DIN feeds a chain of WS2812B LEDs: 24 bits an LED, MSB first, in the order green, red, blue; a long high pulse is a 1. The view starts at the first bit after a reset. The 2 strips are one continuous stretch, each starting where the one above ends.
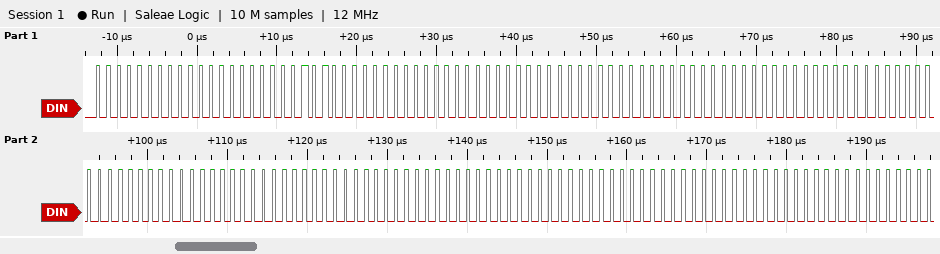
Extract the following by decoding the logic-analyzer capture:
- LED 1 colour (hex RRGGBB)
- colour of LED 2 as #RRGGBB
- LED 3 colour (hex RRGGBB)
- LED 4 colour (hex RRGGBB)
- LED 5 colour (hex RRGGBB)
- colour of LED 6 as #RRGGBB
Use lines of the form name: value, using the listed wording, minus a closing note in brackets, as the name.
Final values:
LED 1 colour: #00000A
colour of LED 2 as #RRGGBB: #000000
LED 3 colour: #000000
LED 4 colour: #000000
LED 5 colour: #000000
colour of LED 6 as #RRGGBB: #000000
